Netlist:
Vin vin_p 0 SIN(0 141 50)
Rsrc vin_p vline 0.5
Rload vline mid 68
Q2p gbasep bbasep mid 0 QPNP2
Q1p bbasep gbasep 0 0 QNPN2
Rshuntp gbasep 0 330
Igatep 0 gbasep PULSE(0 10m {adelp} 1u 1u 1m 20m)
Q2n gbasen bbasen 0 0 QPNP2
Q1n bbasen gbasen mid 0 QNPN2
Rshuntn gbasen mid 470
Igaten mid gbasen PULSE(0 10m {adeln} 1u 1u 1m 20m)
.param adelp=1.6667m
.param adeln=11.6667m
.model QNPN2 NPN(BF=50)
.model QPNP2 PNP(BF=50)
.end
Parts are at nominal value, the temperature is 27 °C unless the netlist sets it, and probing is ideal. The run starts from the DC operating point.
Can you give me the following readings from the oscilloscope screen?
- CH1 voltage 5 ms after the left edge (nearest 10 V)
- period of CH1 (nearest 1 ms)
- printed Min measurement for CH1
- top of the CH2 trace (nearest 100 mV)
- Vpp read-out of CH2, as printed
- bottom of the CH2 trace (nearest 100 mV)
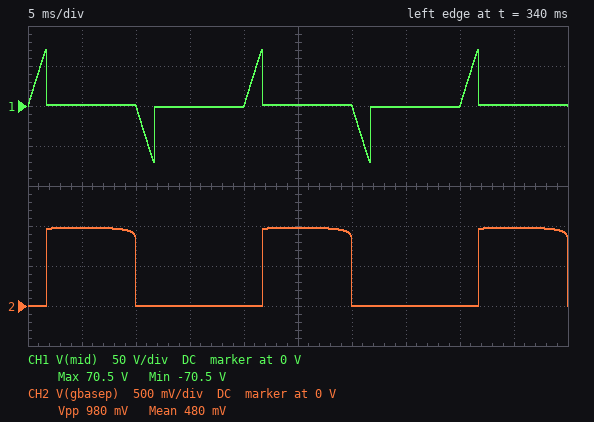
0 V
20 ms
-70.5 V
1.0 V
980 mV
0 V
